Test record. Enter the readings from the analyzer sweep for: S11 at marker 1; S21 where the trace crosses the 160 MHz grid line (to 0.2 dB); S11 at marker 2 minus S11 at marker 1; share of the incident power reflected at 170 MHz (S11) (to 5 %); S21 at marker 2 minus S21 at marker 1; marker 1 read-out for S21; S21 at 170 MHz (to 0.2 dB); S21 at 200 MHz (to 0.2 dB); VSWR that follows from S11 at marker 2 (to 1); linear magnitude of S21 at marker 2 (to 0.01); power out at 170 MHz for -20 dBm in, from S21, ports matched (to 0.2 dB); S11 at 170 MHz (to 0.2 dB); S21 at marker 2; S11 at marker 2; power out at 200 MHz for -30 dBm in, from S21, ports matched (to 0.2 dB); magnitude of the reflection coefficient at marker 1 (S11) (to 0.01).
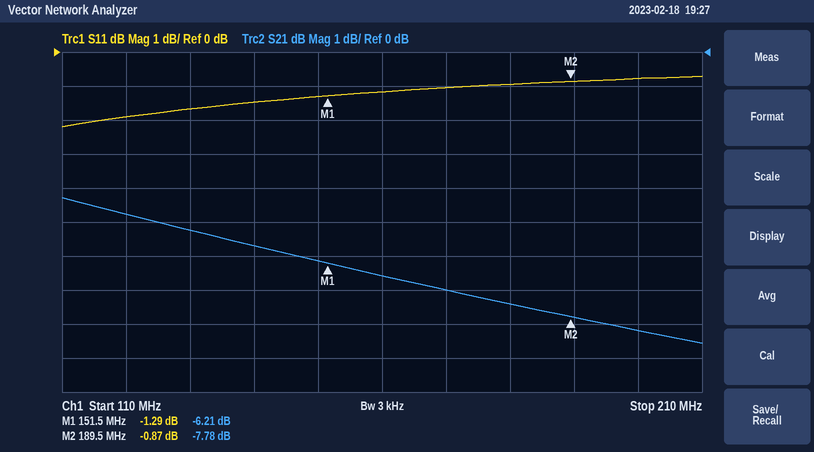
-1.29 dB
-6.6 dB
0.42 dB
80 %
-1.57 dB
-6.21 dB
-7.0 dB
-8.2 dB
20
0.41
-27.0 dBm
-1.0 dB
-7.78 dB
-0.87 dB
-38.2 dBm
0.86
